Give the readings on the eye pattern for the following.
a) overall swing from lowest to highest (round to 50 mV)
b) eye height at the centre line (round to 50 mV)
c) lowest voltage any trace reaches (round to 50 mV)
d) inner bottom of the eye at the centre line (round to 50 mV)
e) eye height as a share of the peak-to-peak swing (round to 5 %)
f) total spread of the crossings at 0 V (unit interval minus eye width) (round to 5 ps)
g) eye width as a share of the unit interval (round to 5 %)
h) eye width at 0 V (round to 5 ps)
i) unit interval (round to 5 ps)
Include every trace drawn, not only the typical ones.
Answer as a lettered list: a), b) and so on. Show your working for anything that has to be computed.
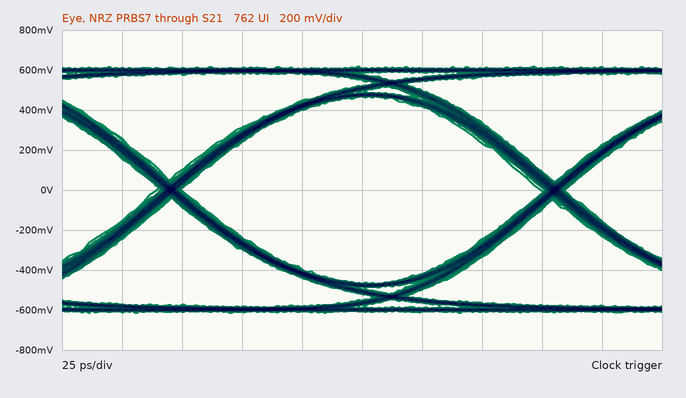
a) 1.25 V
b) 950 mV
c) -600 mV
d) -450 mV
e) 950 mV / 1.25 V ≈ 76.0 %, so 75 % to the nearest 5 %
f) 10 ps
g) 150 ps / 160 ps ≈ 93.8 %, so 95 % to the nearest 5 %
h) 150 ps
i) 160 ps
